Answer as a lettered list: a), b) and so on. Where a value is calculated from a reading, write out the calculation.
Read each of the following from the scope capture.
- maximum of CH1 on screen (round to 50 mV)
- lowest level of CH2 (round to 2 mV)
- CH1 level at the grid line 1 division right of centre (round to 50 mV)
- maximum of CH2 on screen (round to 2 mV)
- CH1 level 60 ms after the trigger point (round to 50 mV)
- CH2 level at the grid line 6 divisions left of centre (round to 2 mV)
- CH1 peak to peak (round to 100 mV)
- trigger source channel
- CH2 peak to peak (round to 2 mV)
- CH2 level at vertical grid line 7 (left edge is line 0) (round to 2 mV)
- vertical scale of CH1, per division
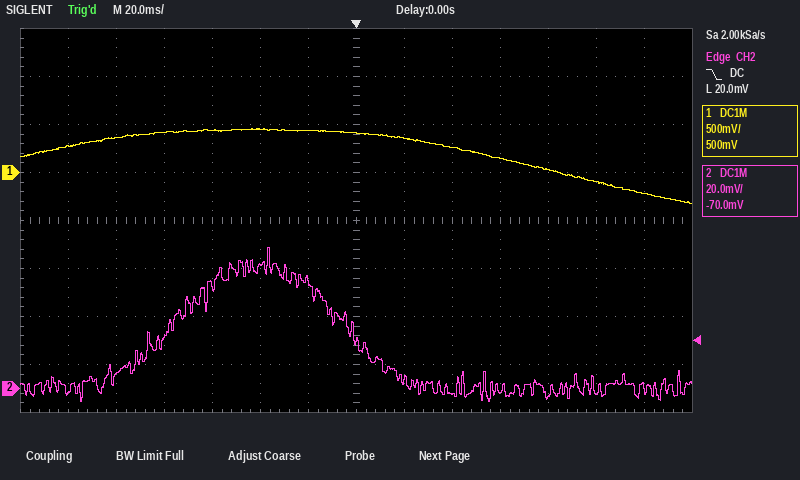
a) 450 mV
b) -6 mV
c) 350 mV
d) 58 mV
e) 150 mV
f) -2 mV
g) 800 mV
h) CH2
i) 58 mV − (-6 mV) = 64 mV
j) 20 mV
k) 500 mV
